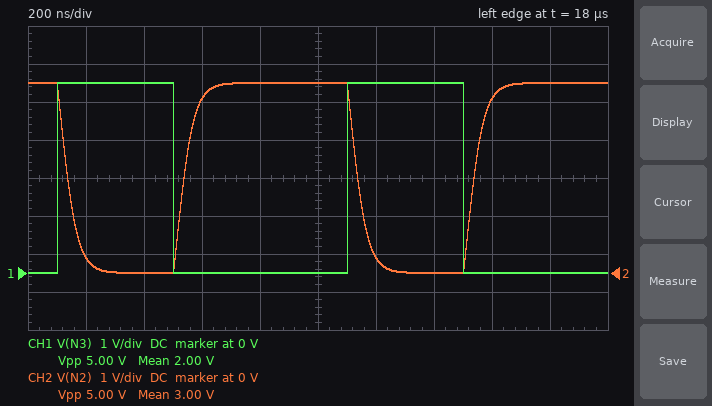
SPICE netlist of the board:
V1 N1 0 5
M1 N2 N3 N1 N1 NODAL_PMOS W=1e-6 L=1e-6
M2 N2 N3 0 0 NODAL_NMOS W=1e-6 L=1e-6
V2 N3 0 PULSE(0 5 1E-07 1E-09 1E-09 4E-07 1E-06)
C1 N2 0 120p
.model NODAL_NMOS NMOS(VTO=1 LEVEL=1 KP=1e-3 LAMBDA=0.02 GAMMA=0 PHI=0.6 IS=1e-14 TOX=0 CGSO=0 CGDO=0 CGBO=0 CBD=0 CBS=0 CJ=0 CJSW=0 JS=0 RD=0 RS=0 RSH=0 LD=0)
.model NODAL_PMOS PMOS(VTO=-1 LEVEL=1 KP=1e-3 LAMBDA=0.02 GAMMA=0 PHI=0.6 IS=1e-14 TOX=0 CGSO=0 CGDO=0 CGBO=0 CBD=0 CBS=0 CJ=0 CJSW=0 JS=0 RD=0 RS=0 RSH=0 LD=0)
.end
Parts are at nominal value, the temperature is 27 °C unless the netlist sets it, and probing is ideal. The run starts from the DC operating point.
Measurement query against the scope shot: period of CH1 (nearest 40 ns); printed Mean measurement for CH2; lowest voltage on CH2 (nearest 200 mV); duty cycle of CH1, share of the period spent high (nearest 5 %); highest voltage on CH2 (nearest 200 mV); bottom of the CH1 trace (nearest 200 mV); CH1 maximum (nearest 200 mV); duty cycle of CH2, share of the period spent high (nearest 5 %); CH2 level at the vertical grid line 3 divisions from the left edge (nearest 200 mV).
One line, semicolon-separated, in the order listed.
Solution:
1.00 µs; 3.00 V; 0 V; 40 %; 5.0 V; 0 V; 5.0 V; 60 %; 4.6 V
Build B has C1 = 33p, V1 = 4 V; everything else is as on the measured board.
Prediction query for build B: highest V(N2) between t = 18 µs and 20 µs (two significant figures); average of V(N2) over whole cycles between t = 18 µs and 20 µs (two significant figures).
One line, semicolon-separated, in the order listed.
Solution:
4.0 V; 2.4 V
